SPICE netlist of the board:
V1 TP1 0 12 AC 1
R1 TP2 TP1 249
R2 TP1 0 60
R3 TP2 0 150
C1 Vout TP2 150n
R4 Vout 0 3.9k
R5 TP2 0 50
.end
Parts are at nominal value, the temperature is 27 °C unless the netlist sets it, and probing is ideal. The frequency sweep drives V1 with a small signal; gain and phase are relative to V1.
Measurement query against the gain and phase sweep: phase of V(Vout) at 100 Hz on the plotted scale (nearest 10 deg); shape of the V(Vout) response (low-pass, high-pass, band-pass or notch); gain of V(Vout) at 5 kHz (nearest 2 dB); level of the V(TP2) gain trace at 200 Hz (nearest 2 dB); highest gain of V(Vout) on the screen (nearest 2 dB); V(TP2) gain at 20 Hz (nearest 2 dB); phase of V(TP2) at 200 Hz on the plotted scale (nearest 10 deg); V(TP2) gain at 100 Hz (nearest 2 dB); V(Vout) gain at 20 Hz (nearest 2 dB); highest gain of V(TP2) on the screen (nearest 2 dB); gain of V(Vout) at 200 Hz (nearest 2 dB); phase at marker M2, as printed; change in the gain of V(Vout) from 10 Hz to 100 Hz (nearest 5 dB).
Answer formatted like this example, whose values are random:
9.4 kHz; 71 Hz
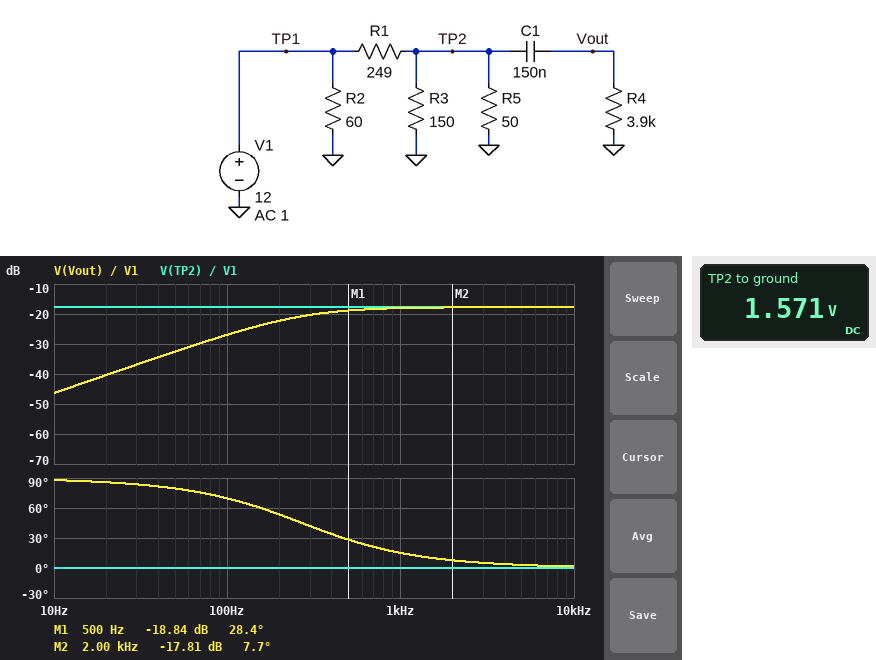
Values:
70 deg; high-pass; -18 dB; -18 dB; -18 dB; -18 dB; 0 deg; -18 dB; -40 dB; -18 dB; -22 dB; 7.7 deg; 20 dB
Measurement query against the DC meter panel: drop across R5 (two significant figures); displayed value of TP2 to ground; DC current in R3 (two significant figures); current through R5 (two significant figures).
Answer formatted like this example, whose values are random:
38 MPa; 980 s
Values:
1.6 V; 1.571 V; 10 mA; 31 mA
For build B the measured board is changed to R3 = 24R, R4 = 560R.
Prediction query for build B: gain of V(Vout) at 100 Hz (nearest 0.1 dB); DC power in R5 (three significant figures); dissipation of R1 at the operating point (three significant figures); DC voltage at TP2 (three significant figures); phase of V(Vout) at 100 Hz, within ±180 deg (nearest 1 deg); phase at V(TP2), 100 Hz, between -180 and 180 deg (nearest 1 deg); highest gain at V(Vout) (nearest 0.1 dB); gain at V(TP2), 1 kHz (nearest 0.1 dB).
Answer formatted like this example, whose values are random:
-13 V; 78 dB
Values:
-49.8 dB; 10.8 mW; 510 mW; 734 mV; 87 deg; 0 deg; -24.5 dB; -24.3 dB
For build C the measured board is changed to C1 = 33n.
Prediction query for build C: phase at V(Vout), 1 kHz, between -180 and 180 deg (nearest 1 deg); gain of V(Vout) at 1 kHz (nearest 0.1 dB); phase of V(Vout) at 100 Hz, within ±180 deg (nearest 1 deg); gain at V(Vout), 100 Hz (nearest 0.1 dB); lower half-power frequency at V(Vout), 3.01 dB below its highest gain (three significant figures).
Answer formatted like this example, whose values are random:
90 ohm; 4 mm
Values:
51 deg; -21.7 dB; 85 deg; -39.5 dB; 1.23 kHz
